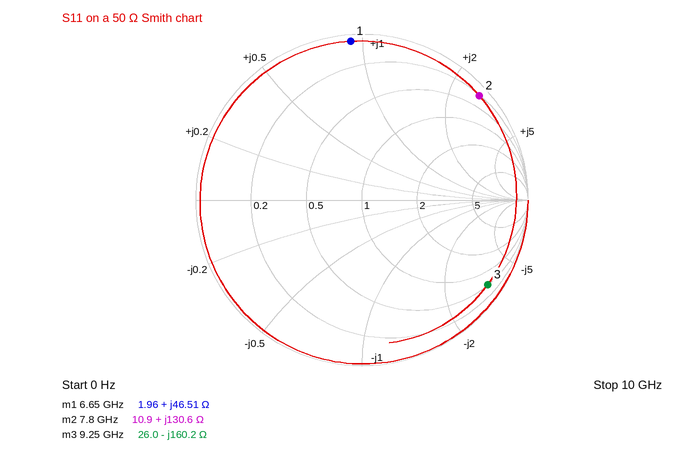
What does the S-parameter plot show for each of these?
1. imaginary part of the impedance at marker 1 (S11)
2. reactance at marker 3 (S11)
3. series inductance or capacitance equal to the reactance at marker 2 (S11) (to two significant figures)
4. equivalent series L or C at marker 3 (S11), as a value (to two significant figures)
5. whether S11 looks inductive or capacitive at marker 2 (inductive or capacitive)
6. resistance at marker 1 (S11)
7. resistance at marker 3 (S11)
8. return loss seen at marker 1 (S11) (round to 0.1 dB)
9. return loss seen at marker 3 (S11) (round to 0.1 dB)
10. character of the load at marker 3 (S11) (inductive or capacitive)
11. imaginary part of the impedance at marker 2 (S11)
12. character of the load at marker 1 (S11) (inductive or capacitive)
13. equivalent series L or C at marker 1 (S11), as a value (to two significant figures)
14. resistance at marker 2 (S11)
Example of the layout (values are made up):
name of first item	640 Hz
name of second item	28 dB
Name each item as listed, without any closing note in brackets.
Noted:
imaginary part of the impedance at marker 1	+46.51 Ω
reactance at marker 3	-160.2 Ω
series inductance or capacitance equal to the reactance at marker 2 (S11)	2.7 nH
equivalent series L or C at marker 3 (S11), as a value	110 fF
whether S11 looks inductive or capacitive at marker 2	inductive
resistance at marker 1	1.96 Ω
resistance at marker 3	26.0 Ω
return loss seen at marker 1 (S11)	0.4 dB
return loss seen at marker 3 (S11)	0.8 dB
character of the load at marker 3 (S11)	capacitive
imaginary part of the impedance at marker 2	+130.6 Ω
character of the load at marker 1 (S11)	inductive
equivalent series L or C at marker 1 (S11), as a value	1.1 nH
resistance at marker 2	10.9 Ω
